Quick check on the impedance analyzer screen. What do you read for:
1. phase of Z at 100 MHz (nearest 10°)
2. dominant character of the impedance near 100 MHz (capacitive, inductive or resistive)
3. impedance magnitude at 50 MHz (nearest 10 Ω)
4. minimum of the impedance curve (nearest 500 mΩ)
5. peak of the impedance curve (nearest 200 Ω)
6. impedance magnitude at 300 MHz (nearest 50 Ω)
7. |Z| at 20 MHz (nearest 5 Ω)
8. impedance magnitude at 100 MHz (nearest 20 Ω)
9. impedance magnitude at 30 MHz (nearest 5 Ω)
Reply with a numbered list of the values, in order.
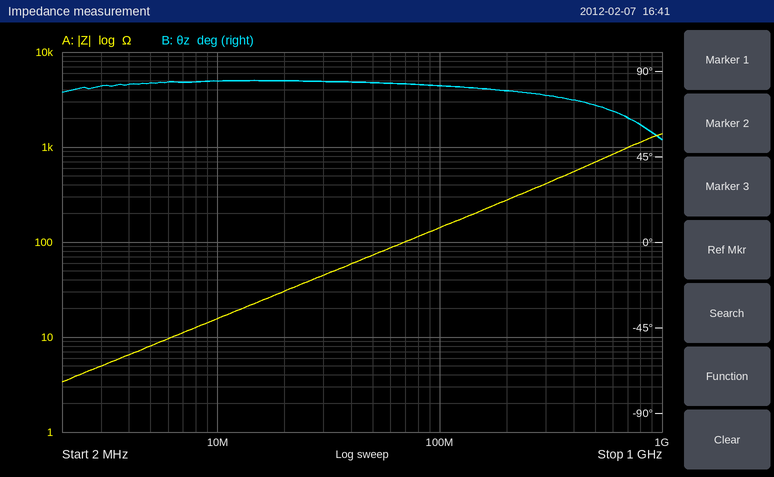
1. 80°
2. inductive
3. 70 Ω
4. 3.5 Ω
5. 1.4 kΩ
6. 400 Ω
7. 30 Ω
8. 140 Ω
9. 45 Ω
